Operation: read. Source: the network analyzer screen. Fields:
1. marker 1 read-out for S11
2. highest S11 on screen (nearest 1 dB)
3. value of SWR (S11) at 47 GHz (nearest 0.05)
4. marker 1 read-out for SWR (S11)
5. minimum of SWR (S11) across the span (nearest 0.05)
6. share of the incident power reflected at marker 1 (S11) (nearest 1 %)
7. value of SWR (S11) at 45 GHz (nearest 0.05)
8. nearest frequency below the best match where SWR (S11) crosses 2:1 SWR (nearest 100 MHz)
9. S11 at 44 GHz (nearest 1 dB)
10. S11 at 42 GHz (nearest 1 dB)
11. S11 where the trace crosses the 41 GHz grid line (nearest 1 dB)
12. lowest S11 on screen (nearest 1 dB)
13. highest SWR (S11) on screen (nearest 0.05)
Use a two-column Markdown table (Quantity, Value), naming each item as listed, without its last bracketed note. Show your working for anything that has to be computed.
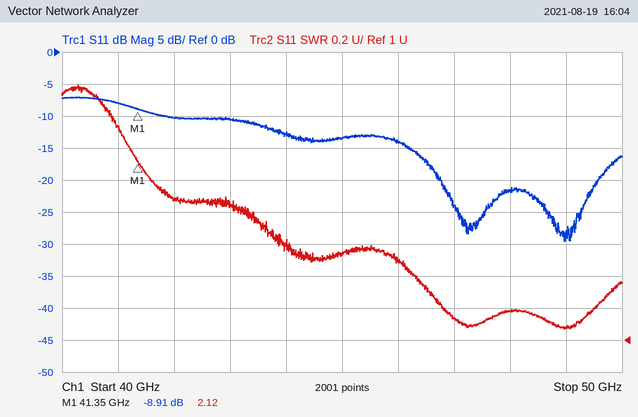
| Quantity | Value |
|---|---|
| marker 1 read-out for S11 | -8.91 dB |
| highest S11 on screen | -7 dB |
| value of SWR (S11) at 47 GHz | 1.15 |
| marker 1 read-out for SWR | 2.12 |
| minimum of SWR (S11) across the span | 1.05 |
| share of the incident power reflected at marker 1 (S11) | 10^(-8.91/10) ≈ 13 % |
| value of SWR (S11) at 45 GHz | 1.55 |
| nearest frequency below the best match where SWR (S11) crosses 2:1 SWR | 41.6 GHz |
| S11 at 44 GHz | -13 dB |
| S11 at 42 GHz | -10 dB |
| S11 where the trace crosses the 41 GHz grid line | -8 dB |
| lowest S11 on screen | -30 dB |
| highest SWR (S11) on screen | 2.60 |
